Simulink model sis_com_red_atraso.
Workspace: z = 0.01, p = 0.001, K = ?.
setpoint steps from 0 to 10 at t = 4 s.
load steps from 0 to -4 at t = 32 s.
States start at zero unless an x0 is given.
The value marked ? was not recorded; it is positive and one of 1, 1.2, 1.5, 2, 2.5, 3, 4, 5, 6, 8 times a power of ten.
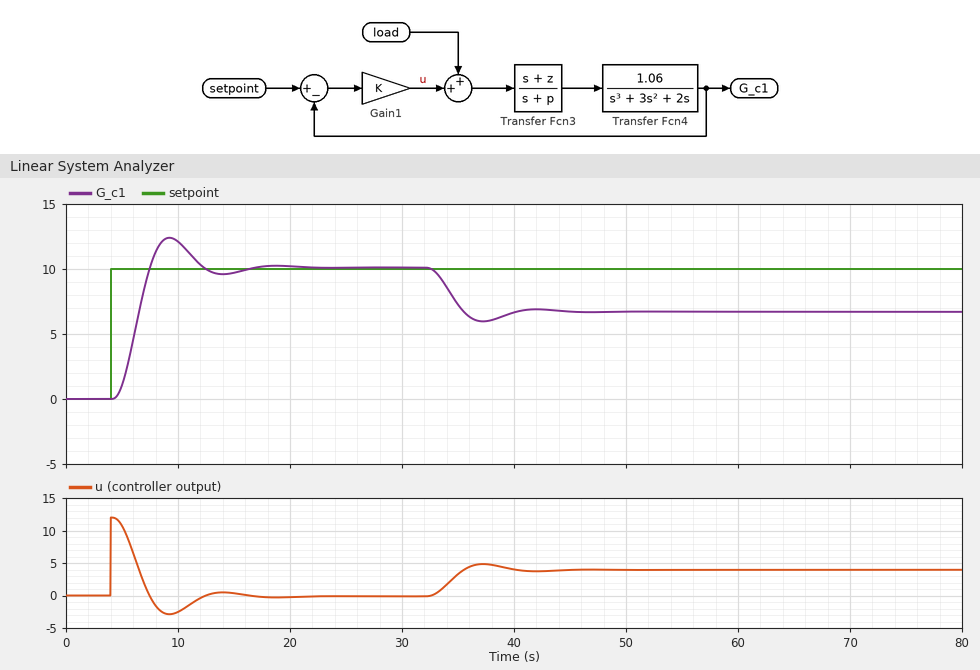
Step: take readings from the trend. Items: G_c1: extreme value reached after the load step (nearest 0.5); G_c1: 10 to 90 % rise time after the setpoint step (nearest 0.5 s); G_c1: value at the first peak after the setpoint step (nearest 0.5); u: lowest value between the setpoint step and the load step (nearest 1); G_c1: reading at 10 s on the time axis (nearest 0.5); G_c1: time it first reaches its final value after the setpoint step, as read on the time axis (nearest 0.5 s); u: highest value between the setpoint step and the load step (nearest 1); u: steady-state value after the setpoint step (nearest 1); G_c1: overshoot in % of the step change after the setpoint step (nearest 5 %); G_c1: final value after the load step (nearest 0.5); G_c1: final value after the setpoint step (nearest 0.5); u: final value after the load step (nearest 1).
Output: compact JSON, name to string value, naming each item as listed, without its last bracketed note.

{"G_c1: extreme value reached after the load step": "6.0", "G_c1: 10 to 90 % rise time after the setpoint step": "2.0 s", "G_c1: value at the first peak after the setpoint step": "12.5", "u: lowest value between the setpoint step and the load step": "-3", "G_c1: reading at 10 s on the time axis": "12.0", "G_c1: time it first reaches its final value after the setpoint step, as read on the time axis": "7.5 s", "u: highest value between the setpoint step and the load step": "12", "u: steady-state value after the setpoint step": "0", "G_c1: overshoot in % of the step change after the setpoint step": "25 %", "G_c1: final value after the load step": "6.5", "G_c1: final value after the setpoint step": "10.0", "u: final value after the load step": "4"}
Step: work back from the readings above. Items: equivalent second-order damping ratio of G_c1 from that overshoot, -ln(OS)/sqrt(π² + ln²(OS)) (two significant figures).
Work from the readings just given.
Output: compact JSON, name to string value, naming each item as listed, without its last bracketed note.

{"equivalent second-order damping ratio of G_c1 from that overshoot, -ln(OS)/sqrt(π² + ln²(OS))": "0.40"}
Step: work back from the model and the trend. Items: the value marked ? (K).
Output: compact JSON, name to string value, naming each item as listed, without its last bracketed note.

{"the value marked ?": "1.2"}
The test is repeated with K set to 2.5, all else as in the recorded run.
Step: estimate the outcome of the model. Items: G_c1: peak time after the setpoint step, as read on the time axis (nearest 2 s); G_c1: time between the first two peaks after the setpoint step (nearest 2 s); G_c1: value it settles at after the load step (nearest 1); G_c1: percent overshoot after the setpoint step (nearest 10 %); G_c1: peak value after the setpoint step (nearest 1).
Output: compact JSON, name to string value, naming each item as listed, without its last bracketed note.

{"G_c1: peak time after the setpoint step, as read on the time axis": "8 s", "G_c1: time between the first two peaks after the setpoint step": "6 s", "G_c1: value it settles at after the load step": "8", "G_c1: percent overshoot after the setpoint step": "50 %", "G_c1: peak value after the setpoint step": "15"}
